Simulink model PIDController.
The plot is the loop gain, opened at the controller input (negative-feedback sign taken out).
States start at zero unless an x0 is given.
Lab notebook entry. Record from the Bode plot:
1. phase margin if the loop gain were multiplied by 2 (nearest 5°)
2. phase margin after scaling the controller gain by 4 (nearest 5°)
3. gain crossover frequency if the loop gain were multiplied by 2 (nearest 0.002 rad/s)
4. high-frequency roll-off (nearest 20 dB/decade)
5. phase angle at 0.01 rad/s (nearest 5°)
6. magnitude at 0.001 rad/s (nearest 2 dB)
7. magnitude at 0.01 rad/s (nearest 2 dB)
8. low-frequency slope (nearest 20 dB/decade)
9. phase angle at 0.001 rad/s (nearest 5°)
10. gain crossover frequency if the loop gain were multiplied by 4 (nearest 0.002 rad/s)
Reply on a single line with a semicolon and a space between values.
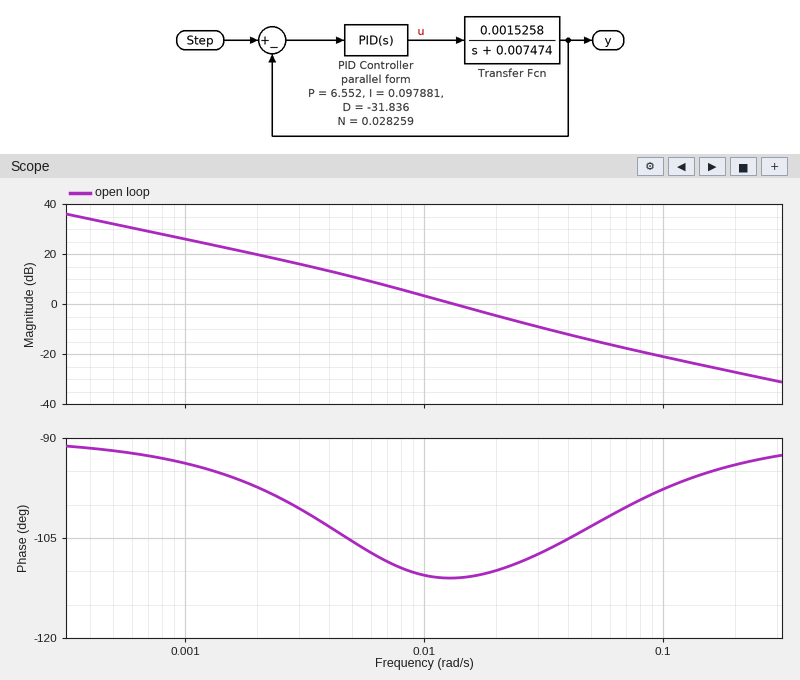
70°; 75°; 0.022 rad/s; -20 dB/decade; -110°; 26 dB; 4 dB; -20 dB/decade; -95°; 0.040 rad/s
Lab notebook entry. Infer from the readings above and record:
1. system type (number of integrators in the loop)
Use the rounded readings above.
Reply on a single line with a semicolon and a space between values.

1
